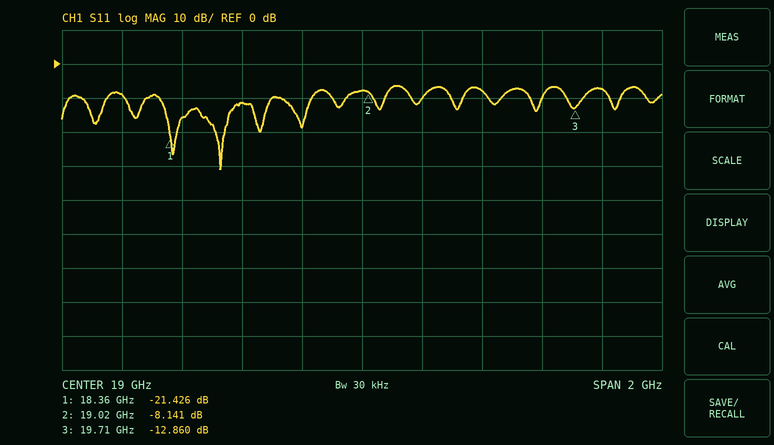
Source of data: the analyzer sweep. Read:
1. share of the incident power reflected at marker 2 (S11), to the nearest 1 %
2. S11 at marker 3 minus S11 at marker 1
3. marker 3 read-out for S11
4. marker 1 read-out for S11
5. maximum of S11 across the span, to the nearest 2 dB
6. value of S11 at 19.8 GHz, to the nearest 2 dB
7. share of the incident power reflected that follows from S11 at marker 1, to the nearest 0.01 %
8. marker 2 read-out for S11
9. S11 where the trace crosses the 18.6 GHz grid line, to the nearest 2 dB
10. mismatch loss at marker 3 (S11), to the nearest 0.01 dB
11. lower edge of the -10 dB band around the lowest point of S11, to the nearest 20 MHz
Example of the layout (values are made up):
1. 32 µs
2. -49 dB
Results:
1. 15 %
2. 8.566 dB
3. -12.860 dB
4. -21.426 dB
5. -6 dB
6. -8 dB
7. 0.72 %
8. -8.141 dB
9. -12 dB
10. 0.23 dB
11. 18.32 GHz
